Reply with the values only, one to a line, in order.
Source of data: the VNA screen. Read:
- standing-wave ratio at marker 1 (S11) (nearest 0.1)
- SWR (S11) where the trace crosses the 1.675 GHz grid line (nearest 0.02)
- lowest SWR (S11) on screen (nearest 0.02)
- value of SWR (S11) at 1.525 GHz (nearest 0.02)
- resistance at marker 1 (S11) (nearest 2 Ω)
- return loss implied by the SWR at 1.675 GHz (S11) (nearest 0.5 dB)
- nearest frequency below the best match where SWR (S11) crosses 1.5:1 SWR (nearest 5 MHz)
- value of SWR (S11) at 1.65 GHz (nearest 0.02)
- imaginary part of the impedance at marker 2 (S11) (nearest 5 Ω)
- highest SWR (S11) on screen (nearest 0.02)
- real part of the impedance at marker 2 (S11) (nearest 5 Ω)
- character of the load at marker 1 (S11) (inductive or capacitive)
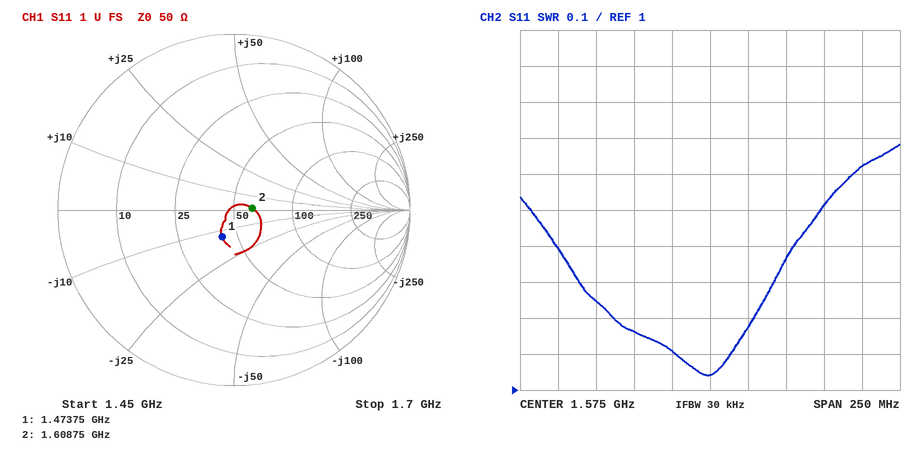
1.4
1.62
1.04
1.16
42 Ω
12.5 dB
1.455 GHz
1.52
0 Ω
1.68
60 Ω
capacitive
